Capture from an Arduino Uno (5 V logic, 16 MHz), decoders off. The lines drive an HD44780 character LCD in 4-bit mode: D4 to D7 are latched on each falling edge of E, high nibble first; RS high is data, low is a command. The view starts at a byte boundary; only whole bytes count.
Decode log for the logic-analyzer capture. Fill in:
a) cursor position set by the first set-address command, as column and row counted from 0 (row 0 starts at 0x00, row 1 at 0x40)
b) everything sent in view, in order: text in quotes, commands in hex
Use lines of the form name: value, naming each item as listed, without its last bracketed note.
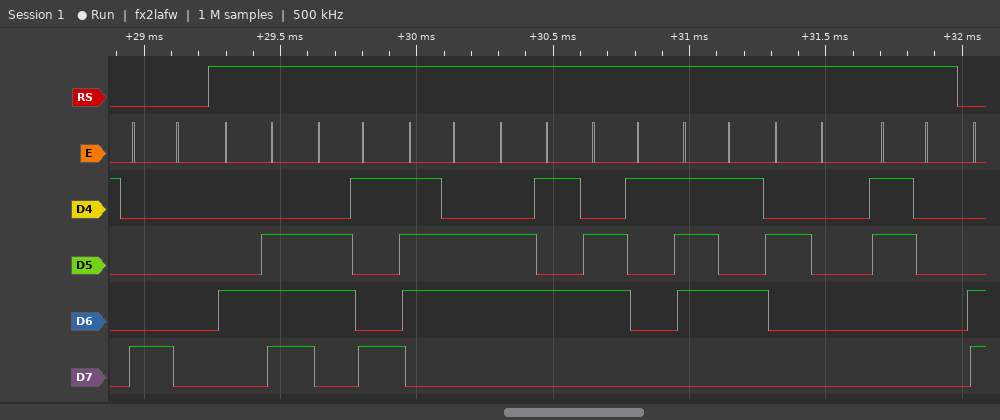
cursor position set by the first set-address command, as column and row counted from 0: column 0, row 0
everything sent in view, in order: text in quotes, commands in hex: 0x80 "Niveau 0"
